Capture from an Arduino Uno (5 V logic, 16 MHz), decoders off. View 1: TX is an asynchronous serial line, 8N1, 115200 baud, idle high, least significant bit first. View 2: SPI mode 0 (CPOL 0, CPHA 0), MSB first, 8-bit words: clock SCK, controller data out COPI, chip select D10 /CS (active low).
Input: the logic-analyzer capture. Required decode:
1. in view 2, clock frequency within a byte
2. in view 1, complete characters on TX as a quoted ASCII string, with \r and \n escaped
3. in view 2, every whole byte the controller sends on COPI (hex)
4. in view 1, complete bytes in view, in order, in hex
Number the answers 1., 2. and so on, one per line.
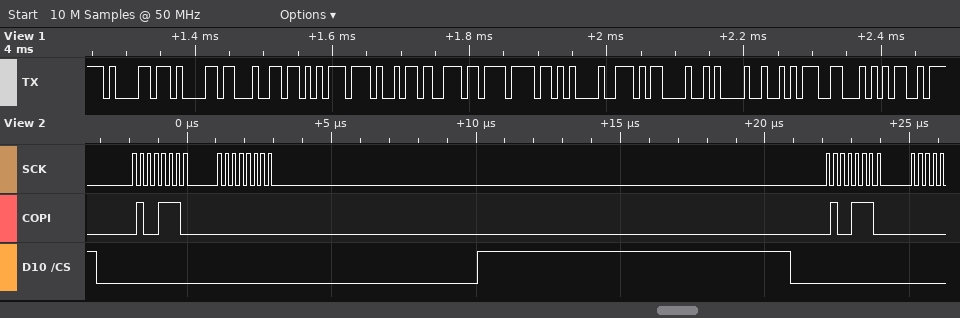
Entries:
1. 4 MHz
2. "aaduino!\r\nRFM"
3. 0x4E 0x00 0x4E
4. 61 61 64 75 69 6E 6F 21 0D 0A 52 46 4D
